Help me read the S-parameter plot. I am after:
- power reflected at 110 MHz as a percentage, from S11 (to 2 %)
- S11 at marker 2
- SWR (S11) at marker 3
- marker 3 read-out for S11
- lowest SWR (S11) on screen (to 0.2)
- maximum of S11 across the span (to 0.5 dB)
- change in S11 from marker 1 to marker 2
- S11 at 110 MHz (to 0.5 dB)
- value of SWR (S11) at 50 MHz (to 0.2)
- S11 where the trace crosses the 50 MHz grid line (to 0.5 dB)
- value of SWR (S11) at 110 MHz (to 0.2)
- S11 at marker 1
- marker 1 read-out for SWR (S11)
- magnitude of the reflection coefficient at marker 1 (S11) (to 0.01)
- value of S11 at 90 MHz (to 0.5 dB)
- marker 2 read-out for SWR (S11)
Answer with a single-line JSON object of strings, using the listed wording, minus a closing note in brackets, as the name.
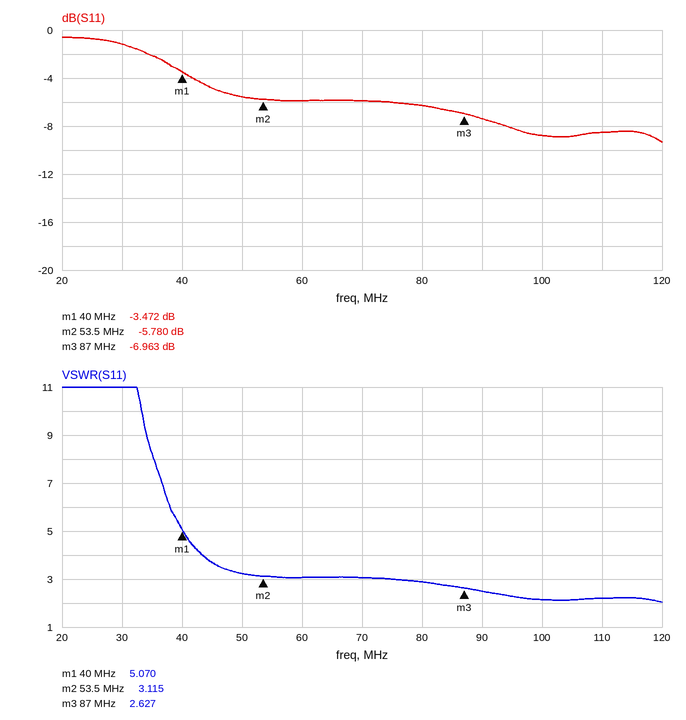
{"power reflected at 110 MHz as a percentage, from S11": "14 %", "S11 at marker 2": "-5.780 dB", "SWR (S11) at marker 3": "2.627", "marker 3 read-out for S11": "-6.963 dB", "lowest SWR (S11) on screen": "2.0", "maximum of S11 across the span": "-0.5 dB", "change in S11 from marker 1 to marker 2": "-2.308 dB", "S11 at 110 MHz": "-8.5 dB", "value of SWR (S11) at 50 MHz": "3.2", "S11 where the trace crosses the 50 MHz grid line": "-5.5 dB", "value of SWR (S11) at 110 MHz": "2.2", "S11 at marker 1": "-3.472 dB", "marker 1 read-out for SWR": "5.070", "magnitude of the reflection coefficient at marker 1 (S11)": "0.67", "value of S11 at 90 MHz": "-7.5 dB", "marker 2 read-out for SWR": "3.115"}
